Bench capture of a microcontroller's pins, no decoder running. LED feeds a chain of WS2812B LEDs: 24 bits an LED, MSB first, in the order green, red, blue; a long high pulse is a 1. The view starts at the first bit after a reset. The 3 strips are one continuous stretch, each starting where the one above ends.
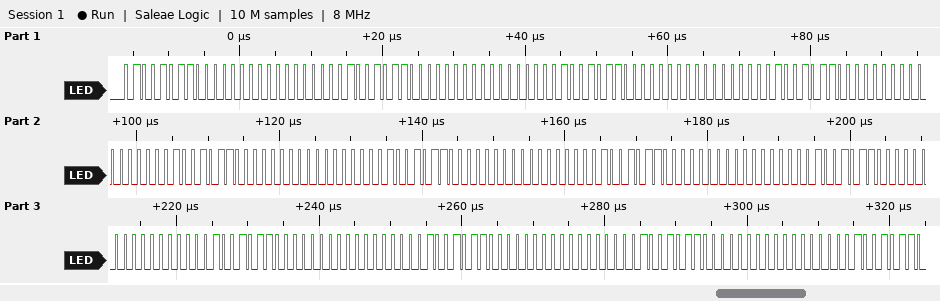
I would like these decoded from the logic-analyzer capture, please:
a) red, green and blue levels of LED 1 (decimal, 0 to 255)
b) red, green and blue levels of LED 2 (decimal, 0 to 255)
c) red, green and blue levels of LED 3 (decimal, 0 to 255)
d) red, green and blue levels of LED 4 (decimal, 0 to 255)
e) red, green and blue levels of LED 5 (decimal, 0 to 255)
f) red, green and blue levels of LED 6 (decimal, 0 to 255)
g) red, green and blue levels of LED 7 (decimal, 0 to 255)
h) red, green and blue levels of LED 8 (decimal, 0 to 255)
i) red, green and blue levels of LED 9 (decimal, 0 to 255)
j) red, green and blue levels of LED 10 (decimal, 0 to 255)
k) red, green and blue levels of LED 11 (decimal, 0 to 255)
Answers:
0, 75, 0
0, 75, 0
0, 75, 0
0, 75, 0
0, 75, 0
0, 75, 0
0, 75, 0
0, 75, 0
0, 75, 0
0, 75, 0
0, 75, 0
